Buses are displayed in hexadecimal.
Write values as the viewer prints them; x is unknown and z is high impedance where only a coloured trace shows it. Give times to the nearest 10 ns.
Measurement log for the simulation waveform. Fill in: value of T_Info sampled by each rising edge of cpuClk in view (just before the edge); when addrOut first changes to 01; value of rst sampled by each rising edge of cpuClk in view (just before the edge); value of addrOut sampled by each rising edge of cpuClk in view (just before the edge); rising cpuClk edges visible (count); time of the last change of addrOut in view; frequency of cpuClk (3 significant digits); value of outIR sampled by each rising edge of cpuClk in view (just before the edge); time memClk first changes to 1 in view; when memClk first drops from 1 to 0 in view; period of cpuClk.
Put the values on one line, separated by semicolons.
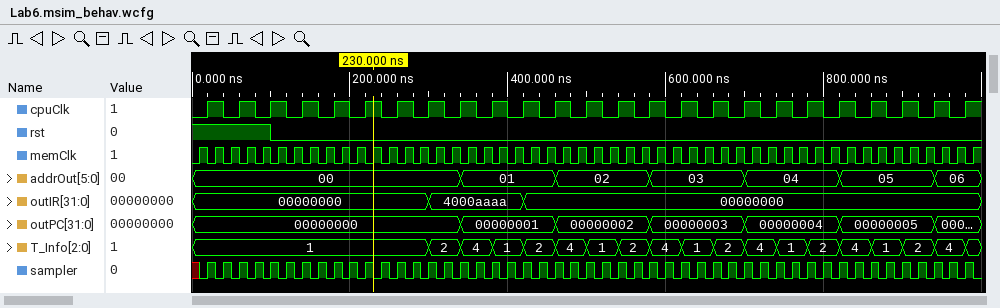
1, 1, 1, 1, 1, 1, 1, 1, 2, 4, 1, 2, 4, 1, 2, 4, 1, 2, 4, 1, 2, 4, 1, 2, 4; 340 ns; 1 1 1 0 0 0 0 0 0 0 0 0 0 0 0 0 0 0 0 0 0 0 0 0 0; 00, 00, 00, 00, 00, 00, 00, 00, 00, 01, 01, 01, 02, 02, 02, 03, 03, 03, 04, 04, 04, 05, 05, 05, 06; 25; 940 ns; 25.0 MHz; 00000000, 00000000, 00000000, 00000000, 00000000, 00000000, 00000000, 00000000, 4000aaaa, 4000aaaa, 4000aaaa, 00000000, 00000000, 00000000, 00000000, 00000000, 00000000, 00000000, 00000000, 00000000, 00000000, 00000000, 00000000, 00000000, 00000000; 10 ns; 20 ns; 40 ns
